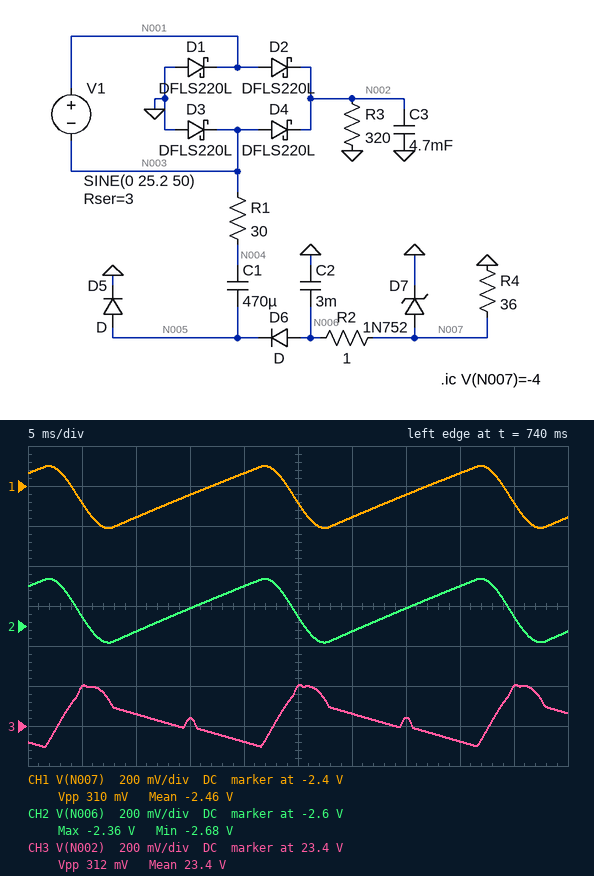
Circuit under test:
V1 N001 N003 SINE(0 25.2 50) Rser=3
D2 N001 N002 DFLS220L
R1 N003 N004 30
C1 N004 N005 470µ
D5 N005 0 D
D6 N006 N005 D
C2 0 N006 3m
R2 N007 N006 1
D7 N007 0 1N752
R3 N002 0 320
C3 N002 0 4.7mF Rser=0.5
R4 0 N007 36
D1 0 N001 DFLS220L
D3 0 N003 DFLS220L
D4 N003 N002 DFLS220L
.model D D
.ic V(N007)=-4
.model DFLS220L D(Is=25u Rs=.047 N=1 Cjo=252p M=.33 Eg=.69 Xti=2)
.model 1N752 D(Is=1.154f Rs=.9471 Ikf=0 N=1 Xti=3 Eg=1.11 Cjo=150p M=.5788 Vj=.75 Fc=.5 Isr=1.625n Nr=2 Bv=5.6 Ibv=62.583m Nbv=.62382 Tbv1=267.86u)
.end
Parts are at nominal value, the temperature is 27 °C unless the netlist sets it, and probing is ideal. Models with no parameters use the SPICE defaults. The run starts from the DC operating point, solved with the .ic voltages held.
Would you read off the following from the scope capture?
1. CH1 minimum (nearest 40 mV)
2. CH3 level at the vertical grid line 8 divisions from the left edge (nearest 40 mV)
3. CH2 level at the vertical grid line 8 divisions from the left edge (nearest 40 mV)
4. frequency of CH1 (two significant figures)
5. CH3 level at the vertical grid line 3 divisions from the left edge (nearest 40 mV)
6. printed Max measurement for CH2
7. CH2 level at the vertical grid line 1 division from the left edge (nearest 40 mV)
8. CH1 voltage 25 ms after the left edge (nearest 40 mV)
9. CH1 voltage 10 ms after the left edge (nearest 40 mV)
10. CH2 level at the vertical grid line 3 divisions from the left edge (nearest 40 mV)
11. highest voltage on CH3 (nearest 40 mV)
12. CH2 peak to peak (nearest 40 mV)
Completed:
-2.60 V
23.32 V
-2.40 V
50 Hz
23.44 V
-2.36 V
-2.56 V
-2.48 V
-2.56 V
-2.52 V
23.60 V
320 mV
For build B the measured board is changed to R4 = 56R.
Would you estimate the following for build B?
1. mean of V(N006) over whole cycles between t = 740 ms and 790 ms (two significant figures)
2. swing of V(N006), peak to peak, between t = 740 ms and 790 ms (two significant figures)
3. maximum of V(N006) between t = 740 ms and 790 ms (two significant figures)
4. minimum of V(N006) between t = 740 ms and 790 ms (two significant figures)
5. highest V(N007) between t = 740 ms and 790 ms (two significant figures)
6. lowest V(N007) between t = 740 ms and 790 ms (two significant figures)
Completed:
-3.6 V
300 mV
-3.5 V
-3.8 V
-3.4 V
-3.7 V
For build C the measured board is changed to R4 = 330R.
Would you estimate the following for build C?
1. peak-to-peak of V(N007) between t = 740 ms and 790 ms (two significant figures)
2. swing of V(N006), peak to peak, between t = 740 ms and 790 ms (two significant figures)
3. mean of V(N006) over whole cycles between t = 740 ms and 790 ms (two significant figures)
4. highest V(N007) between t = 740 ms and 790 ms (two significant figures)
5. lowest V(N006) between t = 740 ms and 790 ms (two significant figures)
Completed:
140 mV
240 mV
-5.7 V
-5.6 V
-5.8 V
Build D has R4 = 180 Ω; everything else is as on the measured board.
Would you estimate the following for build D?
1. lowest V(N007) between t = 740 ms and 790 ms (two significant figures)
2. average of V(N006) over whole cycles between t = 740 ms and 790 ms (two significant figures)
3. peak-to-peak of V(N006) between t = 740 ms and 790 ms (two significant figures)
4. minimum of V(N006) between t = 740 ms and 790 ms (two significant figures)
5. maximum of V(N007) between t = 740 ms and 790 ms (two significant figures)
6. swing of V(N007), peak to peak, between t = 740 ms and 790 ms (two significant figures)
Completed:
-5.7 V
-5.6 V
240 mV
-5.8 V
-5.5 V
170 mV
